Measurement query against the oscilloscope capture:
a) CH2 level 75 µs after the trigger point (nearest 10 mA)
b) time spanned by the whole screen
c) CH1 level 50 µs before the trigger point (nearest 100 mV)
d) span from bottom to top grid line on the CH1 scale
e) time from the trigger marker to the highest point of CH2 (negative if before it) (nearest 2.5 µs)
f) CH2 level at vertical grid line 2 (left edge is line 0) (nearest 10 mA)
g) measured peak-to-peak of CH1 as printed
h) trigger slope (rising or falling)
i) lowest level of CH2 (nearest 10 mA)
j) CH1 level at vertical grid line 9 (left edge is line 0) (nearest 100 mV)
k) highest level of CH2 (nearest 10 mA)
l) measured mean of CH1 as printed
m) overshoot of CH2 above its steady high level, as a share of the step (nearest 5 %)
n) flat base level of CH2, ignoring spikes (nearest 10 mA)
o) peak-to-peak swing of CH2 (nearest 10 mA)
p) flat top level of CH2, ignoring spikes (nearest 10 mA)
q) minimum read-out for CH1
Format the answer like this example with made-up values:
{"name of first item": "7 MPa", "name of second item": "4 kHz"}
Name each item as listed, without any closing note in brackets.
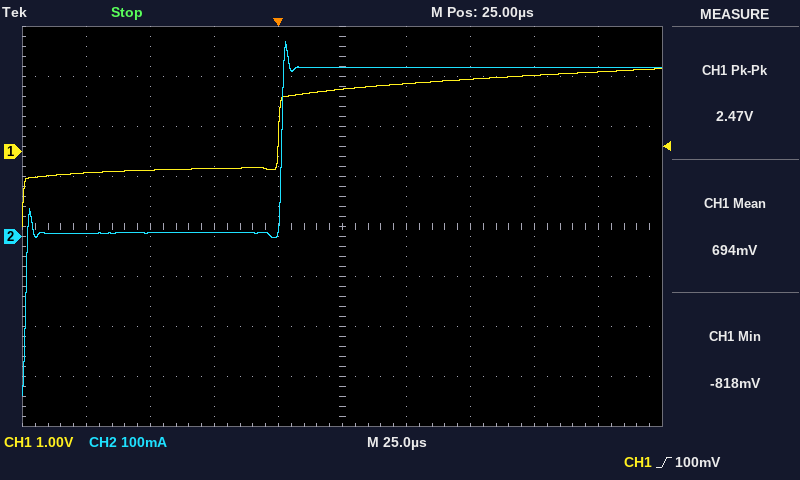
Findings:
{"CH2 level 75 µs after the trigger point": "340 mA", "time spanned by the whole screen": "250 µs", "CH1 level 50 µs before the trigger point": "-400 mV", "span from bottom to top grid line on the CH1 scale": "8 V", "time from the trigger marker to the highest point of CH2 (negative if before it)": "+2.5 µs", "CH2 level at vertical grid line 2 (left edge is line 0)": "10 mA", "measured peak-to-peak of CH1 as printed": "2.47 V", "trigger slope": "rising", "lowest level of CH2": "-320 mA", "CH1 level at vertical grid line 9 (left edge is line 0)": "1.6 V", "highest level of CH2": "390 mA", "measured mean of CH1 as printed": "694 mV", "overshoot of CH2 above its steady high level, as a share of the step": "15 %", "flat base level of CH2, ignoring spikes": "10 mA", "peak-to-peak swing of CH2": "710 mA", "flat top level of CH2, ignoring spikes": "340 mA", "minimum read-out for CH1": "-818 mV"}
